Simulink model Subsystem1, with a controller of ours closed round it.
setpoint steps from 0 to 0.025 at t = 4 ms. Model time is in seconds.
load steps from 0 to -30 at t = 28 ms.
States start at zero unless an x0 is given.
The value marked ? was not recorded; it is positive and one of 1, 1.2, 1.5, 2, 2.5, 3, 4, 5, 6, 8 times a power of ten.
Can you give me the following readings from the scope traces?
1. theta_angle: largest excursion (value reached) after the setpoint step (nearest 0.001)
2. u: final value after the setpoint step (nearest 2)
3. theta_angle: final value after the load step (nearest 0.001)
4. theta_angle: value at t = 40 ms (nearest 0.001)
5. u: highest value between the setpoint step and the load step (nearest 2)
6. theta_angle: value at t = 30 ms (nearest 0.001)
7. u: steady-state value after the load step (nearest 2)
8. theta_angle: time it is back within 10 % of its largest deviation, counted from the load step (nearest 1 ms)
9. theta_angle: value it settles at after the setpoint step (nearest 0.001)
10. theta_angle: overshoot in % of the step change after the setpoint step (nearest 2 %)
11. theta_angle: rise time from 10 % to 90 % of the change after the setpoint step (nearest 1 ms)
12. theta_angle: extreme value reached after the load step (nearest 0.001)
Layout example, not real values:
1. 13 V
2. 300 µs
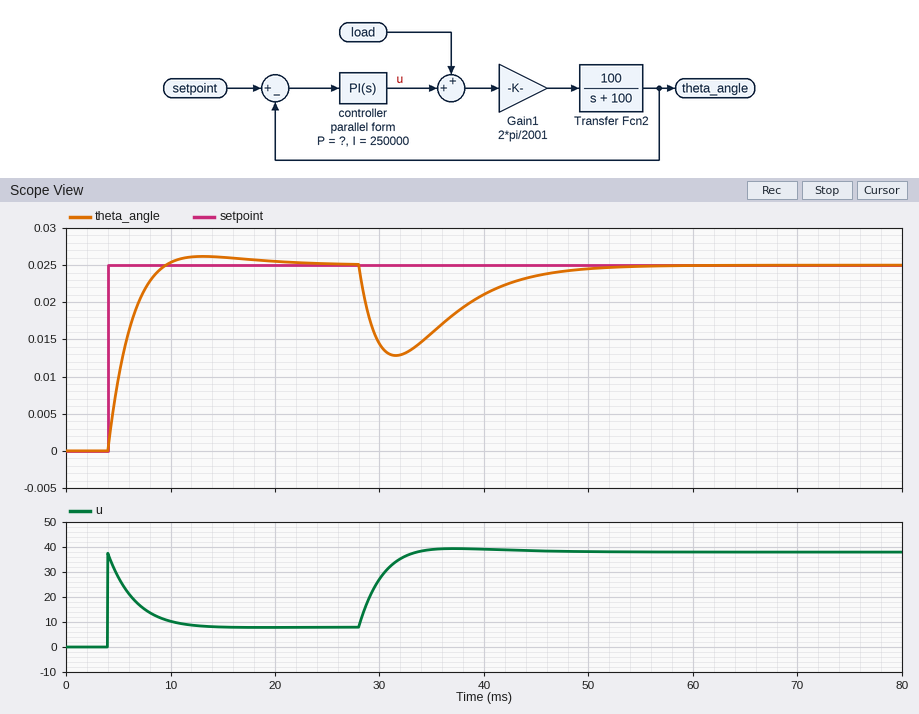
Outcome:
1. 0.026
2. 8
3. 0.025
4. 0.021
5. 38
6. 0.014
7. 38
8. 18 ms
9. 0.025
10. 4 %
11. 4 ms
12. 0.013
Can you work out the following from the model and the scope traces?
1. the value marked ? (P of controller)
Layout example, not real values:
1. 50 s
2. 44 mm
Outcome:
1. 1500
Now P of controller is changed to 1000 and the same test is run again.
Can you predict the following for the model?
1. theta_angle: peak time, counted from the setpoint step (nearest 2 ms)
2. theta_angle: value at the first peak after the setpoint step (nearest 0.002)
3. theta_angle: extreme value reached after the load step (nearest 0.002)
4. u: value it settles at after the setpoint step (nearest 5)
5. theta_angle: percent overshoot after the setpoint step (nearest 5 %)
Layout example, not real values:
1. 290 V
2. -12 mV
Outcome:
1. 10 ms
2. 0.028
3. 0.010
4. 10
5. 10 %
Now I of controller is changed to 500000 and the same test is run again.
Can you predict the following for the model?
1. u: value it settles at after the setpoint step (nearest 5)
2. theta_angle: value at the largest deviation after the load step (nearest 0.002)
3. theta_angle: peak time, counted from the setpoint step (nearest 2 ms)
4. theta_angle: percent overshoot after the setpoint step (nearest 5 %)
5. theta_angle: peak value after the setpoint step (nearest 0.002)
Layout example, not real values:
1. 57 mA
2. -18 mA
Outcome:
1. 10
2. 0.014
3. 6 ms
4. 15 %
5. 0.028
